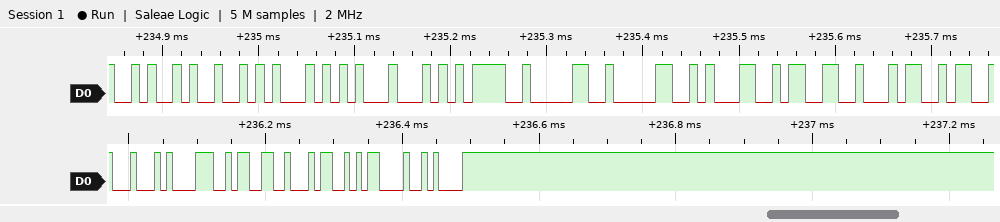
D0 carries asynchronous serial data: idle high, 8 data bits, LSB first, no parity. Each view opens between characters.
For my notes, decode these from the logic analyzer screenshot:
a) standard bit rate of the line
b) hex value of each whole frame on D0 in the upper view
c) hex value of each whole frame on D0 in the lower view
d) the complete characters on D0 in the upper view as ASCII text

115200 baud
4A, 52, 54, 44, 3D, 30, 30, 31, 33, 34
44, 38, 33, 34, 0D, 0A
"JRTD=00134"
